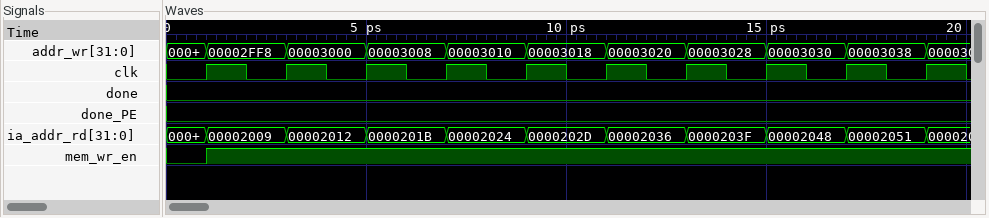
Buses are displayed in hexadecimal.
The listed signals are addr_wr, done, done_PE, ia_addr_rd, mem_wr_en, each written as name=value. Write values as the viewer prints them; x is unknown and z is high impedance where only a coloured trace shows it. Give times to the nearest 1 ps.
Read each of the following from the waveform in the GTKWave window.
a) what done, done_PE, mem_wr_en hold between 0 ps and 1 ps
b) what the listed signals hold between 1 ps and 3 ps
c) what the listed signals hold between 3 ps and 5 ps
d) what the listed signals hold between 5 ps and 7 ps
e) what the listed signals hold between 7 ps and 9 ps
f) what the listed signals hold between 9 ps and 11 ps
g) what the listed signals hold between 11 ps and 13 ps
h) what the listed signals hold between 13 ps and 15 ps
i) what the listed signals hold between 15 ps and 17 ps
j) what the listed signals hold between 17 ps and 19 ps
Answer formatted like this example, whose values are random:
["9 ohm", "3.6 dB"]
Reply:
["done=0, done_PE=0, mem_wr_en=0", "addr_wr=00002FF8, done=0, done_PE=0, ia_addr_rd=00002009, mem_wr_en=1", "addr_wr=00003000, done=0, done_PE=0, ia_addr_rd=00002012, mem_wr_en=1", "addr_wr=00003008, done=0, done_PE=0, ia_addr_rd=0000201B, mem_wr_en=1", "addr_wr=00003010, done=0, done_PE=0, ia_addr_rd=00002024, mem_wr_en=1", "addr_wr=00003018, done=0, done_PE=0, ia_addr_rd=0000202D, mem_wr_en=1", "addr_wr=00003020, done=0, done_PE=0, ia_addr_rd=00002036, mem_wr_en=1", "addr_wr=00003028, done=0, done_PE=0, ia_addr_rd=0000203F, mem_wr_en=1", "addr_wr=00003030, done=0, done_PE=0, ia_addr_rd=00002048, mem_wr_en=1", "addr_wr=00003038, done=0, done_PE=0, ia_addr_rd=00002051, mem_wr_en=1"]
